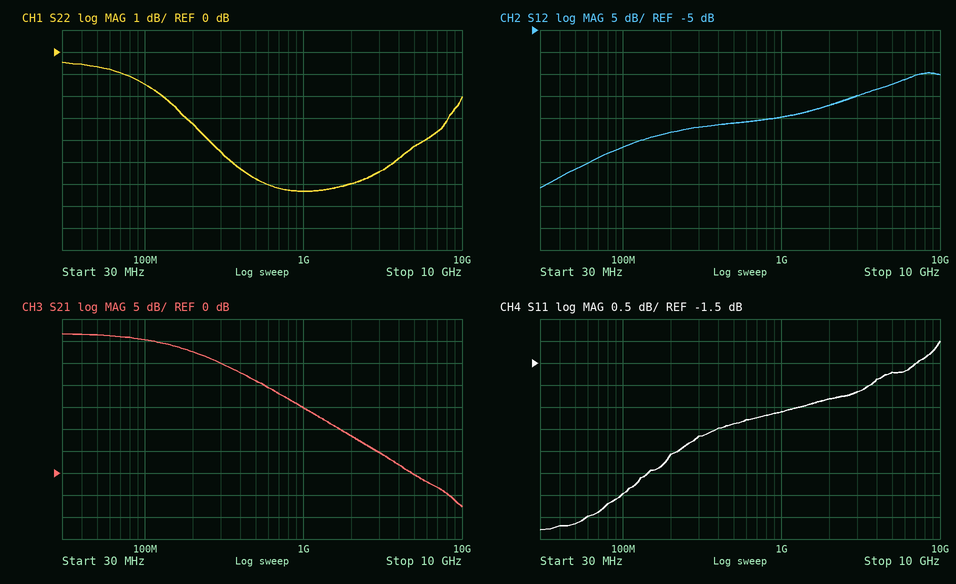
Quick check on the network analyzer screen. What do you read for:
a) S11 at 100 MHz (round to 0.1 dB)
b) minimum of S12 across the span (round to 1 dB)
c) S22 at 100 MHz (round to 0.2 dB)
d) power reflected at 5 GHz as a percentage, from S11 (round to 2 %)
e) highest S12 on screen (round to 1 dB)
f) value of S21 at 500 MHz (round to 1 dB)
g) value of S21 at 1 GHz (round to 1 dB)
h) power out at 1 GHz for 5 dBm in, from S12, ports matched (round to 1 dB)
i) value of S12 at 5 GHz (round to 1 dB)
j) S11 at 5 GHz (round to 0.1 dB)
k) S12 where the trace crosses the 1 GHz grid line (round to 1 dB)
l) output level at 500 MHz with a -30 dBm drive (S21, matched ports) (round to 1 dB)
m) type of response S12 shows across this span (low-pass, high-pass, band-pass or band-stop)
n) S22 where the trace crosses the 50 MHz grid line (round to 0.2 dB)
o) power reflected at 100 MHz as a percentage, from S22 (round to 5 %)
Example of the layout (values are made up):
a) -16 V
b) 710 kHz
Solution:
a) -4.5 dB
b) -41 dB
c) -1.4 dB
d) 68 %
e) -15 dB
f) 21 dB
g) 15 dB
h) -20 dBm
i) -17 dB
j) -1.7 dB
k) -25 dB
l) -9 dBm
m) high-pass
n) -0.6 dB
o) 70 %
